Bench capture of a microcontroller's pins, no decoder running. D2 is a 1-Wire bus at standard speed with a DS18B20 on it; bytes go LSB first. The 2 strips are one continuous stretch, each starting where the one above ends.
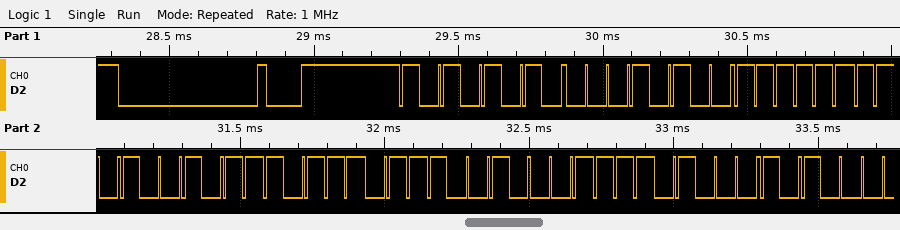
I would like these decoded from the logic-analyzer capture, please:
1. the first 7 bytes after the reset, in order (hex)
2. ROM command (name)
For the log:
55 28 FF D2 DD 89 17
Match ROM
